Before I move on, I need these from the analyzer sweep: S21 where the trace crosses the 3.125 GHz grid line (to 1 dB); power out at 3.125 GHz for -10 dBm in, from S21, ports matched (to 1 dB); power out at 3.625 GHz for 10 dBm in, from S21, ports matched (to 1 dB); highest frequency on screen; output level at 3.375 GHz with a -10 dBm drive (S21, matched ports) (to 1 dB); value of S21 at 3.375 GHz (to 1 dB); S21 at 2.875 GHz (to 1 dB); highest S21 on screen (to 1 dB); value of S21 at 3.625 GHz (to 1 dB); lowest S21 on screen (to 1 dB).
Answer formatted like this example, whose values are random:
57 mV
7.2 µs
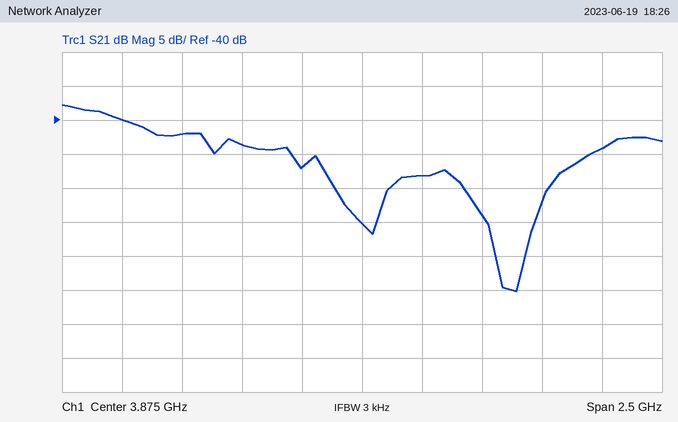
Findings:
-42 dB
-52 dBm
-37 dBm
5.125 GHz
-54 dBm
-44 dB
-40 dB
-38 dB
-47 dB
-65 dB
